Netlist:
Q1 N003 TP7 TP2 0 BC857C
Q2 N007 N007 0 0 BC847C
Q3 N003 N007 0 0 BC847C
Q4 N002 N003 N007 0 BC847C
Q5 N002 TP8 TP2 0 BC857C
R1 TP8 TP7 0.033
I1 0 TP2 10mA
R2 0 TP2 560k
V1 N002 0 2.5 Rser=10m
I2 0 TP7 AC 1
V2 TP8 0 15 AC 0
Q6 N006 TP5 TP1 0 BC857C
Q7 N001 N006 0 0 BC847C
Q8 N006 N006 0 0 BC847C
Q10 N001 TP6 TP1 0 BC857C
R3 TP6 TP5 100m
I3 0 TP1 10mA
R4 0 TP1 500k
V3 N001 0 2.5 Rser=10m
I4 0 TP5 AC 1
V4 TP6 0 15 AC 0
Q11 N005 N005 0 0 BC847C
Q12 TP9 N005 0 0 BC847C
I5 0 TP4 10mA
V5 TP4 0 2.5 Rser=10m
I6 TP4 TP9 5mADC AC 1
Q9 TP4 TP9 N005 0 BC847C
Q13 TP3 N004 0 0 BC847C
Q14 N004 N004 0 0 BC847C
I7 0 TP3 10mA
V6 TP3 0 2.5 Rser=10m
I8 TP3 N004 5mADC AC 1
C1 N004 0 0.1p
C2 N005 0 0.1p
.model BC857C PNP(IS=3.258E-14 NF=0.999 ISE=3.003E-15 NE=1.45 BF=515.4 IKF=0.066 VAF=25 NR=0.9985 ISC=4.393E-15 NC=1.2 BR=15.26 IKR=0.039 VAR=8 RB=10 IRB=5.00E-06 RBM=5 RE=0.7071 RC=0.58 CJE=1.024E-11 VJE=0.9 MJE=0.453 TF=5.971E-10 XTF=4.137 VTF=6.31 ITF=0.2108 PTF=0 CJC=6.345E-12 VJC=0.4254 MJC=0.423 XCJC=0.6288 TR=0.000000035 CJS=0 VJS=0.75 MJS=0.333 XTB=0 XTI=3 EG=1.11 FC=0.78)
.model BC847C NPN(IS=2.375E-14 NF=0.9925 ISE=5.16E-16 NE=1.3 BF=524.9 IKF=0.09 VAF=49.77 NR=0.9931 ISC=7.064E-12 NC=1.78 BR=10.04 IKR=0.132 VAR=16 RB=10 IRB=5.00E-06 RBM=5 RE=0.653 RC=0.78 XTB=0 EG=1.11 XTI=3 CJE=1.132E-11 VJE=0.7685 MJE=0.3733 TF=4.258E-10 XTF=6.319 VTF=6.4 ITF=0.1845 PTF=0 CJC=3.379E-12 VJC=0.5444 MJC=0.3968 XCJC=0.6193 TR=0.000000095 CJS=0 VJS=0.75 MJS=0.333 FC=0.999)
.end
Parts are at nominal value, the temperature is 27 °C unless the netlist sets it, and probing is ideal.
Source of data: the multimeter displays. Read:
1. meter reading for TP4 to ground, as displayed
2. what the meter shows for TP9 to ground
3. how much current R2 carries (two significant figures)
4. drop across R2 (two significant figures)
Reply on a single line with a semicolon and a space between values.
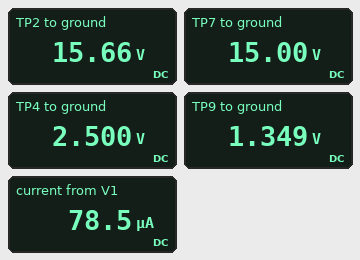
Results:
2.500 V; 1.349 V; 28 µA; 16 V
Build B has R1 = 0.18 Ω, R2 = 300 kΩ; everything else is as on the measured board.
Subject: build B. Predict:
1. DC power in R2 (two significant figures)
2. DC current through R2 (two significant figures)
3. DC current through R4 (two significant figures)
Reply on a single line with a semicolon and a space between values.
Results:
820 µW; 52 µA; 31 µA
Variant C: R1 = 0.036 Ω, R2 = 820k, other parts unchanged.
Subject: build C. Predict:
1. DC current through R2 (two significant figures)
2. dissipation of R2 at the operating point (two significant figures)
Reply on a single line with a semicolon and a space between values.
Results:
19 µA; 300 µW
